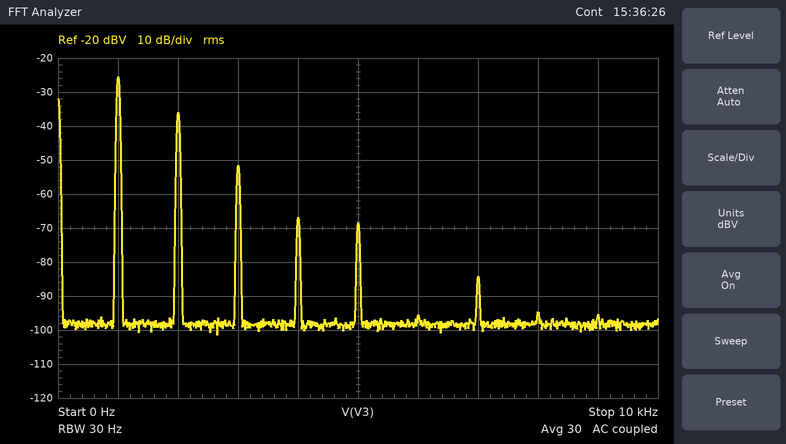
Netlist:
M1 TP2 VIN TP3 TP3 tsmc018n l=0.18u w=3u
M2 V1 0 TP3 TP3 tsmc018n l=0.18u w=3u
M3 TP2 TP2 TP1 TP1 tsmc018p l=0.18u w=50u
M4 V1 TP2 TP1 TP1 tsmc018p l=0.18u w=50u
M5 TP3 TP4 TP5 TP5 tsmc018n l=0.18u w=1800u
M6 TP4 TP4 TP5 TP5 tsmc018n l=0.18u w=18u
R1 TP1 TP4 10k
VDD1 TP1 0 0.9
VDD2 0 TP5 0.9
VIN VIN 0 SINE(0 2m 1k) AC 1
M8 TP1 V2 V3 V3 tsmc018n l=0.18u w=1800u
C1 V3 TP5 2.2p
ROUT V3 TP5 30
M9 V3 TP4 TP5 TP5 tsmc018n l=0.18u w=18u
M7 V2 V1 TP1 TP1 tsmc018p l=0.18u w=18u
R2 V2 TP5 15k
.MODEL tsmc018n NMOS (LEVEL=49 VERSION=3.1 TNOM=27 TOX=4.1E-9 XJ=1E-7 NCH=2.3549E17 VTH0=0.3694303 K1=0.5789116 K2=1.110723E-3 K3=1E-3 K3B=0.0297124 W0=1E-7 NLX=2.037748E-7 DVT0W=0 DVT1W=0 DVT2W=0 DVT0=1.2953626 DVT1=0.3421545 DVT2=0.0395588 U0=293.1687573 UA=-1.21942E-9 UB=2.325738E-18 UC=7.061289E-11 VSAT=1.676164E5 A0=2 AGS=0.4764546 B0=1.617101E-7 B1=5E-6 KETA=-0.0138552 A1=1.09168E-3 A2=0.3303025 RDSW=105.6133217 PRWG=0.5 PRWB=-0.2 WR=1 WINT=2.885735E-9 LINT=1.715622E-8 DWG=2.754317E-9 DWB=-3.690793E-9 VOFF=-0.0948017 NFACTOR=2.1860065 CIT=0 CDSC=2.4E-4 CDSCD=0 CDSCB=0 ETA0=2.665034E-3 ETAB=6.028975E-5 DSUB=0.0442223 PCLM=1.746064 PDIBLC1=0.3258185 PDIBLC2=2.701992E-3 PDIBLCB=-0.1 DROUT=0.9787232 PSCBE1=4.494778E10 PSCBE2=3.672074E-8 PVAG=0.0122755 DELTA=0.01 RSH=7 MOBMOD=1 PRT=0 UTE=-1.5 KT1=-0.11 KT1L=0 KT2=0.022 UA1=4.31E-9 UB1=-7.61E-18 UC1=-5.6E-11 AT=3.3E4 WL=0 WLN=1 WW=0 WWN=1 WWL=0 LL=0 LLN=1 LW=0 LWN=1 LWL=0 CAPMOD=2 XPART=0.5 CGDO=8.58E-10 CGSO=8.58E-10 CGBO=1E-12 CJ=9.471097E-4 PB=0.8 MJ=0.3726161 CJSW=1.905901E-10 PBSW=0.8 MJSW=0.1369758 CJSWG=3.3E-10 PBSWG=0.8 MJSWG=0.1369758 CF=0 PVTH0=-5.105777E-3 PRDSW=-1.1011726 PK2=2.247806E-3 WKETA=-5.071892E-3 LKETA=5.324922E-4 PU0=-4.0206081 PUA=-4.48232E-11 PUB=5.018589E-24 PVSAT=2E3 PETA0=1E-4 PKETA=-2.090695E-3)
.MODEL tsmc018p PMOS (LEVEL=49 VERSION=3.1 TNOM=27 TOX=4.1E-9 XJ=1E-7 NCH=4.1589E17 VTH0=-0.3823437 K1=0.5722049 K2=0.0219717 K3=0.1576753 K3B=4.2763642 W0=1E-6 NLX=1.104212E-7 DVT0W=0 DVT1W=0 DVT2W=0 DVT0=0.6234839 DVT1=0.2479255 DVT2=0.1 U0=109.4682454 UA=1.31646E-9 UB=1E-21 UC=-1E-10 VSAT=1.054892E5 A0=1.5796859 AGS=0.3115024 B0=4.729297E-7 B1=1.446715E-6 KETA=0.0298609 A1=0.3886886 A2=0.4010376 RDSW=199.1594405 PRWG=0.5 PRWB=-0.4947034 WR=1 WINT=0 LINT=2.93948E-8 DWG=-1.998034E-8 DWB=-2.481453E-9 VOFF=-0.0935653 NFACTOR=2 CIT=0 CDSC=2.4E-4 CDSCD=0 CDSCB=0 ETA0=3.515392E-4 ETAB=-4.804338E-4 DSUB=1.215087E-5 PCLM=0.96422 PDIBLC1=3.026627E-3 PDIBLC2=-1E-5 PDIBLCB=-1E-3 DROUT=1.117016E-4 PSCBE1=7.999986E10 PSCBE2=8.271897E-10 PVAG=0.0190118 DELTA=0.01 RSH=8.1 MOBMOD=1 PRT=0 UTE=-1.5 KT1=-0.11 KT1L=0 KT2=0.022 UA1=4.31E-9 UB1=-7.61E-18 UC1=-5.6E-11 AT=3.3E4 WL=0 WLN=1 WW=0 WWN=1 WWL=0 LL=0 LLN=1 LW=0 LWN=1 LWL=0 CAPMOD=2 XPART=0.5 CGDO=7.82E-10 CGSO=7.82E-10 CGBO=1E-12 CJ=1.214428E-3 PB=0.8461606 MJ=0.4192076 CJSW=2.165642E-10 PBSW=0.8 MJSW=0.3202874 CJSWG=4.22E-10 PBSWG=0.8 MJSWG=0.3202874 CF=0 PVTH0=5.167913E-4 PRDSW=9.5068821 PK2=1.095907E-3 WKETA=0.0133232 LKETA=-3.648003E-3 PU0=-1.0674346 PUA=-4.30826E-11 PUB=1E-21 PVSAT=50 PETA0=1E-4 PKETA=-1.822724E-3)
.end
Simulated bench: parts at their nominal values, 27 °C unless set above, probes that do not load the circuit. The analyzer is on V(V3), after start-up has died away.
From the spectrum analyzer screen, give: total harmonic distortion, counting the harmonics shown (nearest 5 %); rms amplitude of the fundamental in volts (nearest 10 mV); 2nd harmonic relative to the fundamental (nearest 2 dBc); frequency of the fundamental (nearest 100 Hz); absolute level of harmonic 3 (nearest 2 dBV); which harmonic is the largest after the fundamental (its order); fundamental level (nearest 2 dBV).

30 %
50 mV
-10 dBc
1.0 kHz
-52 dBV
2
-26 dBV
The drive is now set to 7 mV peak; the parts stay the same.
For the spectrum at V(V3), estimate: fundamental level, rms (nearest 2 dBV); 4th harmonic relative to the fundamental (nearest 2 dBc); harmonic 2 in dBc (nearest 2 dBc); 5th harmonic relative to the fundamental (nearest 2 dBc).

-12 dBV
-22 dBc
-8 dBc
-32 dBc
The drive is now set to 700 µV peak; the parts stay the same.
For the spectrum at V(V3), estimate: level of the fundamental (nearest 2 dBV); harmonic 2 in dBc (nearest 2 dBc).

-36 dBV
-18 dBc
